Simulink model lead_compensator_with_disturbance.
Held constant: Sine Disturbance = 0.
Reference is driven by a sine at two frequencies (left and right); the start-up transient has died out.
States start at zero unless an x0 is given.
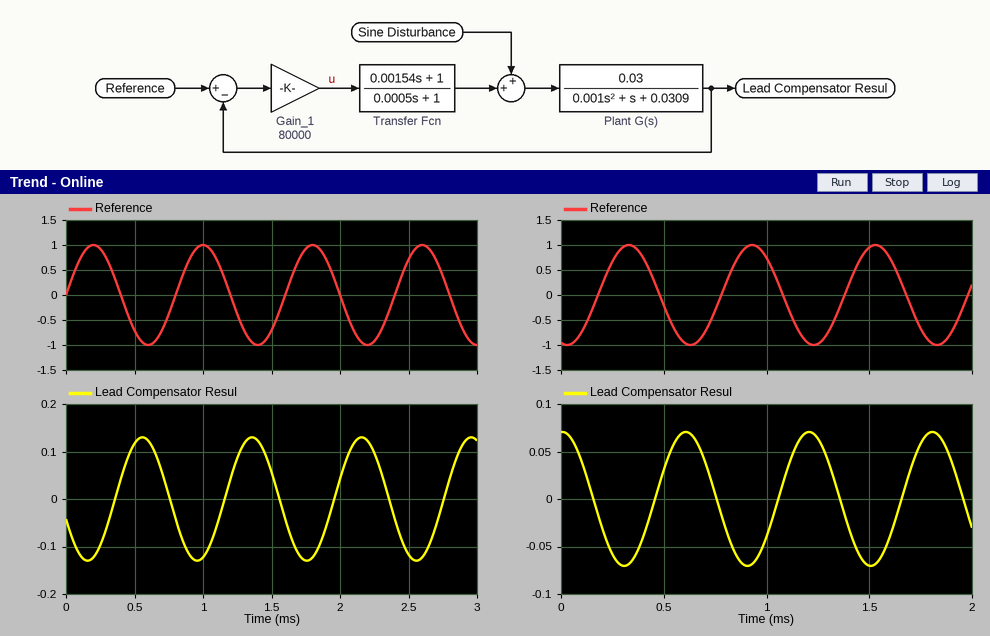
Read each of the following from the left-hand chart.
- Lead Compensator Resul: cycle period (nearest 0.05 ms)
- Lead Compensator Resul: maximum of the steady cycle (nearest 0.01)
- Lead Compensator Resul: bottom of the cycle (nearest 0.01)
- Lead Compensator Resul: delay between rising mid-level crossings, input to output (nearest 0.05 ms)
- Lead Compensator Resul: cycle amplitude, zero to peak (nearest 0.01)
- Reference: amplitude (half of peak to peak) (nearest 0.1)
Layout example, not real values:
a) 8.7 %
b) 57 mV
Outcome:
a) 0.80 ms
b) 0.13
c) -0.13
d) 0.35 ms
e) 0.13
f) 1.0
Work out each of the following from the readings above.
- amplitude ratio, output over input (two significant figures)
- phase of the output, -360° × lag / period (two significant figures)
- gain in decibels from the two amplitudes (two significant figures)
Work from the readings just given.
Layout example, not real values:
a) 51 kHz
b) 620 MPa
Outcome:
a) 0.13
b) -160°
c) -18 dB
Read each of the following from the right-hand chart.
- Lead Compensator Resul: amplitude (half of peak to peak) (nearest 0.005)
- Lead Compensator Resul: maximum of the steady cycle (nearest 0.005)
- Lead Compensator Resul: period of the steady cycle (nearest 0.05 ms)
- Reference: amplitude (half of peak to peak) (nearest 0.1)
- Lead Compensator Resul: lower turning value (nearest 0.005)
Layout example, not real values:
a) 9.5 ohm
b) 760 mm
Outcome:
a) 0.070
b) 0.070
c) 0.60 ms
d) 1.0
e) -0.070
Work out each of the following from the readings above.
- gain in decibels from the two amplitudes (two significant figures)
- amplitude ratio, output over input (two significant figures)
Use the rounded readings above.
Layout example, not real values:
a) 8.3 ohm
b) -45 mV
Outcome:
a) -23 dB
b) 0.070
